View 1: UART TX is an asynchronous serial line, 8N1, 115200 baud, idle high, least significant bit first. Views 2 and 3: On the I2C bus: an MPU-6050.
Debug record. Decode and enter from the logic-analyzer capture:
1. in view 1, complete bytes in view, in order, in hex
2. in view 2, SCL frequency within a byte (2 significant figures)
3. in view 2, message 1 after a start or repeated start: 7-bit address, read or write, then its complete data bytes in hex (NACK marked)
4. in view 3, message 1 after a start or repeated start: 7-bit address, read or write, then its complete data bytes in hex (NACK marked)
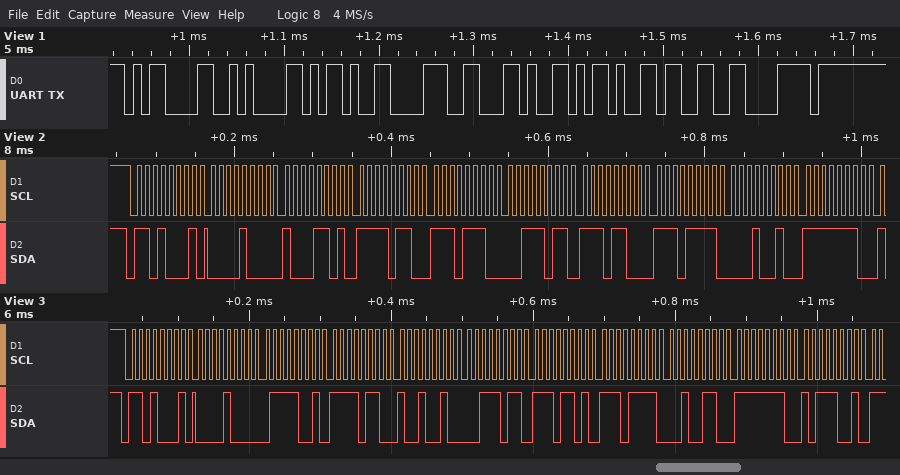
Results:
0x0D 0x0A 0x2D 0x38 0x2C 0x2D 0x33 0x78
100 kHz
0x68 read: 08 8D F6 EE 3B EC EF 12 FE
0x68 read: 08 79 F6 92 3B ED EF 26 FE B9
